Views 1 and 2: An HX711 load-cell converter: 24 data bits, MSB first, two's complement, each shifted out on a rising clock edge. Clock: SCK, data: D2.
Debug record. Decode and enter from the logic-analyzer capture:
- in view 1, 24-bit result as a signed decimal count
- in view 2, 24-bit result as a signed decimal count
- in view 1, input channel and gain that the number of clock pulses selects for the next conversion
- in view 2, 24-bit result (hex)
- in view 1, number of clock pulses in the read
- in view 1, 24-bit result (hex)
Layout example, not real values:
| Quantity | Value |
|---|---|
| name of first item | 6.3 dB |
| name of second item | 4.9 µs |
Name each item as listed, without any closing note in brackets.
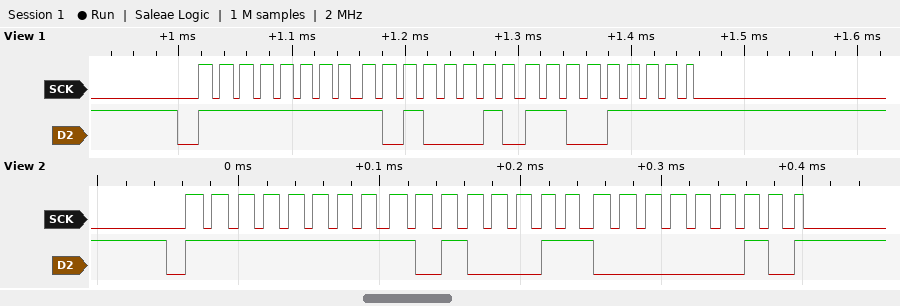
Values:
| Quantity | Value |
|---|---|
| in view 1, 24-bit result as a signed decimal count | -23857 |
| in view 2, 24-bit result as a signed decimal count | -23806 |
| in view 1, input channel and gain that the number of clock pulses selects for the next conversion | channel A, gain 128 |
| in view 2, 24-bit result | 0xFFA302 |
| in view 1, number of clock pulses in the read | 25 |
| in view 1, 24-bit result | 0xFFA2CF |
